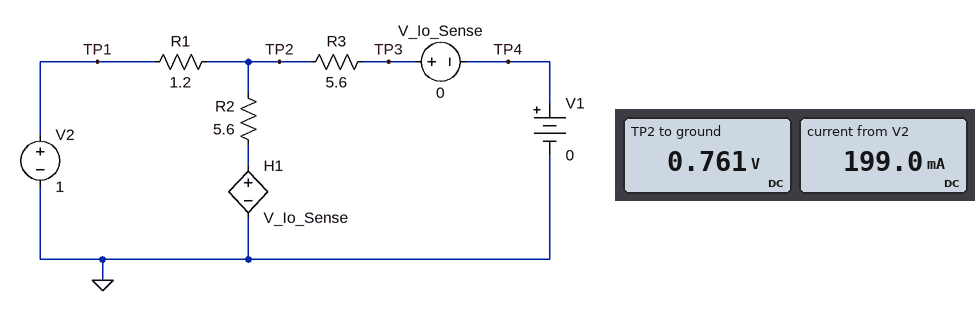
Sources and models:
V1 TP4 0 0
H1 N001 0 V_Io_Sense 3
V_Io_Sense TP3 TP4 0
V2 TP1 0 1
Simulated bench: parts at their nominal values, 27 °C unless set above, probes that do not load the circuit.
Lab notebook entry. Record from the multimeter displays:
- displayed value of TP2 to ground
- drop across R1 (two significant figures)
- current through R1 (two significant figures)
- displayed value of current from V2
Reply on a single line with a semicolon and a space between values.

0.761 V; 240 mV; 200 mA; 199.0 mA
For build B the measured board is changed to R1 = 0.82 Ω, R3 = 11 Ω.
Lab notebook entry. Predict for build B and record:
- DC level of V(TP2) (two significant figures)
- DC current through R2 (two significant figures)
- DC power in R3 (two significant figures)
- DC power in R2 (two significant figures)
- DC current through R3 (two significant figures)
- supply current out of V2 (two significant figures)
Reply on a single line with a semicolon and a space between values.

850 mV; 110 mA; 65 mW; 68 mW; 77 mA; 190 mA
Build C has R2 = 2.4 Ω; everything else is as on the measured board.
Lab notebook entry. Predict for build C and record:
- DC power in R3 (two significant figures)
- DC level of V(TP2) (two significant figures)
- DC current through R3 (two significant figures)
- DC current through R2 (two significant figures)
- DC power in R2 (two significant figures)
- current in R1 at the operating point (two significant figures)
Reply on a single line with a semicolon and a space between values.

85 mW; 690 mV; 120 mA; 130 mA; 43 mW; 260 mA
